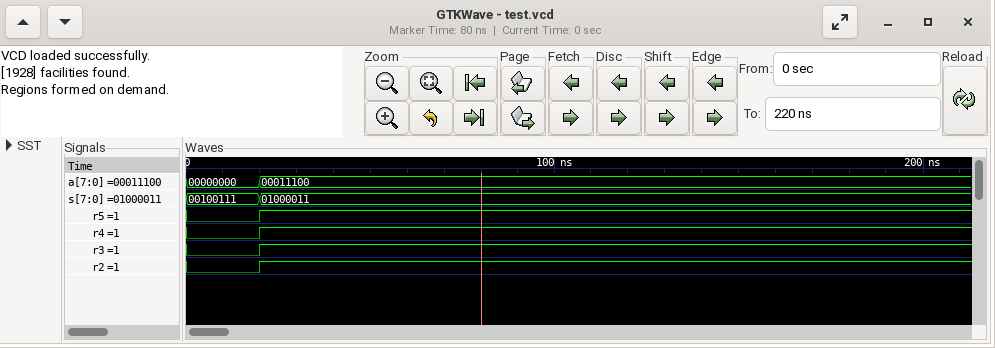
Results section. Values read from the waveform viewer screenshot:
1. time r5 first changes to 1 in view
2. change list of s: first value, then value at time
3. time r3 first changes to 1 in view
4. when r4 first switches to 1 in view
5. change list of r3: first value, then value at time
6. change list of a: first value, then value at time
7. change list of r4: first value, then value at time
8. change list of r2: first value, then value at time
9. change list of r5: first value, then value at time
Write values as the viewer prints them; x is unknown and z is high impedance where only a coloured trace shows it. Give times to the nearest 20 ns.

20 ns
00100111, 01000011 at 20 ns
20 ns
20 ns
0, 1 at 20 ns
00000000, 00011100 at 20 ns
0, 1 at 20 ns
0, 1 at 20 ns
0, 1 at 20 ns
